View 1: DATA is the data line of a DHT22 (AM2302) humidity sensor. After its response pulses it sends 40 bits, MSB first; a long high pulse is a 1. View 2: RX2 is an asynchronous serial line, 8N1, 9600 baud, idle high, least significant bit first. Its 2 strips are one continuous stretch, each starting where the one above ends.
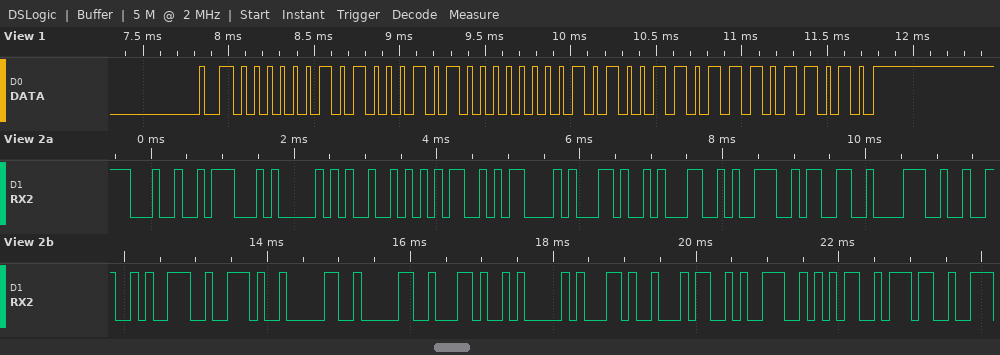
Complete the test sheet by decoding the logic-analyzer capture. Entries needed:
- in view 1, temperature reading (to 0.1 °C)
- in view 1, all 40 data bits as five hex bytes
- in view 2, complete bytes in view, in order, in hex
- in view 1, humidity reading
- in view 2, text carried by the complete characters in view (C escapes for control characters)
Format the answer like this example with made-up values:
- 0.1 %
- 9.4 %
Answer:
- 33.3 °C
- 02 8A 01 4D DA
- 24 47 50 52 4D 43 2C 31 39 33 38 32 39 2E 30 30 2C 41 2C 34 39 35 37
- 65.0 %
- "$GPRMC,193829.00,A,4957"
